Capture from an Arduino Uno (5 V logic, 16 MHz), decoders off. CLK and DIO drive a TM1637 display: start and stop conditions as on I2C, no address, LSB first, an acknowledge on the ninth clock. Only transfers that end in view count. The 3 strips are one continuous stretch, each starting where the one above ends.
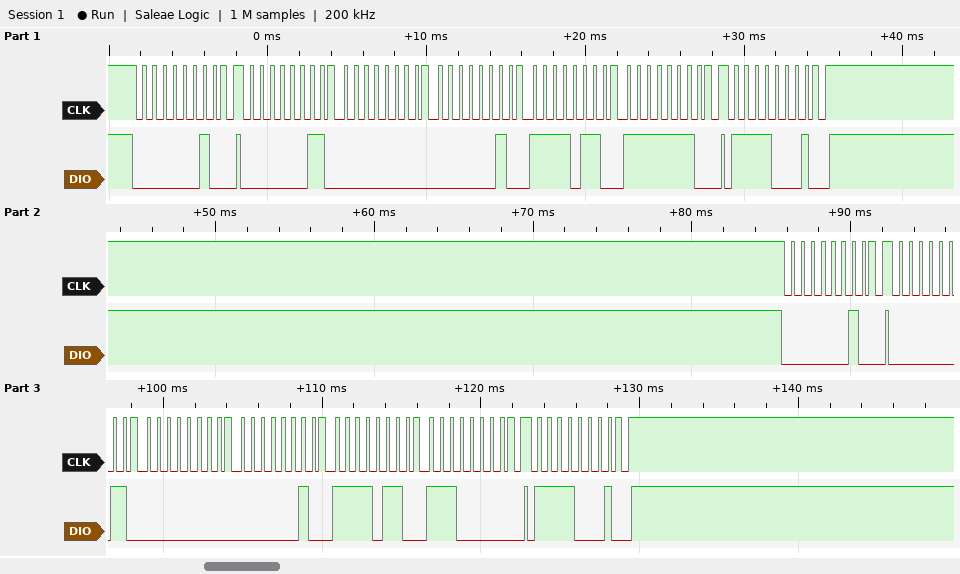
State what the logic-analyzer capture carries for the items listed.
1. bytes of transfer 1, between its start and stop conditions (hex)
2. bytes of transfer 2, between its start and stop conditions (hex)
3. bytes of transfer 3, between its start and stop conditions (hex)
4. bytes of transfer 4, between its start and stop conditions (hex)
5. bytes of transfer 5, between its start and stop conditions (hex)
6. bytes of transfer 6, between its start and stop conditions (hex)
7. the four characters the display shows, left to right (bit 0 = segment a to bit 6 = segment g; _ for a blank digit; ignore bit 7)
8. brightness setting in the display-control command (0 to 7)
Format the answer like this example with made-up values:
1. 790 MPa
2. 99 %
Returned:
1. 40
2. C0 00 40 6F 7F
3. 8F
4. 40
5. C0 00 40 6F 07
6. 8F
7. _-97
8. 7
